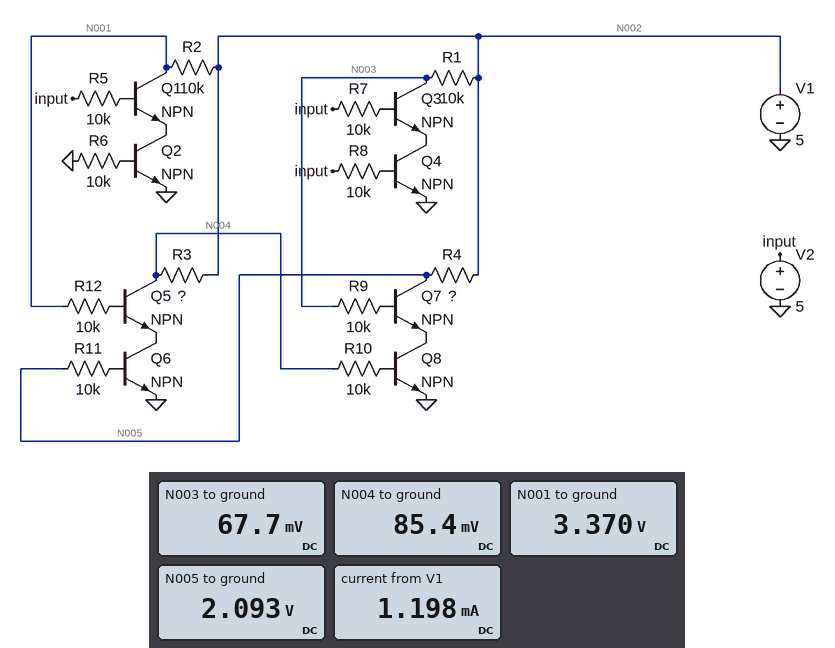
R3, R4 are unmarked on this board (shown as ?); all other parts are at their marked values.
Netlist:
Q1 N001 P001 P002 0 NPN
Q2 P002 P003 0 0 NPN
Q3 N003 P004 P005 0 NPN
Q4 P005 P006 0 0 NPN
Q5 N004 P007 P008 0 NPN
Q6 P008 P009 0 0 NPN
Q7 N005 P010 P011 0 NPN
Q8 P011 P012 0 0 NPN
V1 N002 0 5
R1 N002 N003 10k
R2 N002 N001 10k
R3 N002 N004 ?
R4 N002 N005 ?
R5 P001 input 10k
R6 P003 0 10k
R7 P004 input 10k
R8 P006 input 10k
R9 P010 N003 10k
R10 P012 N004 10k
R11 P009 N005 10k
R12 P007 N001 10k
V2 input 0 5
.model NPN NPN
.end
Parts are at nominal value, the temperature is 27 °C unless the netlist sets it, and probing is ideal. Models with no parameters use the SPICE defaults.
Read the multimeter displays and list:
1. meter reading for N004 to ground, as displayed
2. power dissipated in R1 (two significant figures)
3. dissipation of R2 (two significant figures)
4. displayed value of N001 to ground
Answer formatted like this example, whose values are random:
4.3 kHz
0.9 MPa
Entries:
85.4 mV
2.4 mW
270 µW
3.370 V
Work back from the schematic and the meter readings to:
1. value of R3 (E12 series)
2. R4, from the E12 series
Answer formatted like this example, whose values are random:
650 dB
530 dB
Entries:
12 kΩ
22 kΩ
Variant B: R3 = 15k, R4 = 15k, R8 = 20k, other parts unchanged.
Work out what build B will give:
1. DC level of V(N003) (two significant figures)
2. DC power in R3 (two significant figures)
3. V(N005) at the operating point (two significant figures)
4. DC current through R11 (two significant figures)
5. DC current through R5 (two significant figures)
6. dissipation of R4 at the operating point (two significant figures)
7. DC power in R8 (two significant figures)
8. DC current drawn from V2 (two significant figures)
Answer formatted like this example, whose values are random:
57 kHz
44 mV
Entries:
79 mV
1.6 mW
2.5 V
170 µA
92 µA
430 µW
890 µW
720 µA
